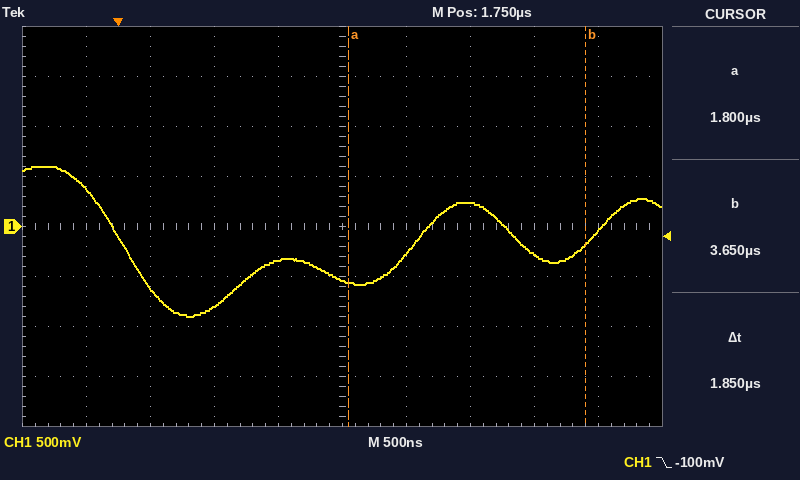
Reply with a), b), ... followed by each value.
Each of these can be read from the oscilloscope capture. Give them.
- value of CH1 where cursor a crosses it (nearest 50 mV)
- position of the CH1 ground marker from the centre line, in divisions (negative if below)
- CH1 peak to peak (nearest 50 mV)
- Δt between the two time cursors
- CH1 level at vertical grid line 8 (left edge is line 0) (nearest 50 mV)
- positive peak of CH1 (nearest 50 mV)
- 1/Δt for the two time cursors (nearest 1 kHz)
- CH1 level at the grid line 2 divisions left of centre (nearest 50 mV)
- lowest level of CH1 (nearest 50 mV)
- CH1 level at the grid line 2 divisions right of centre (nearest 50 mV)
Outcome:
a) -550 mV
b) 0.0 div
c) 1.50 V
d) 1.85 µs
e) -300 mV
f) 600 mV
g) 541 kHz
h) -800 mV
i) -900 mV
j) 250 mV
